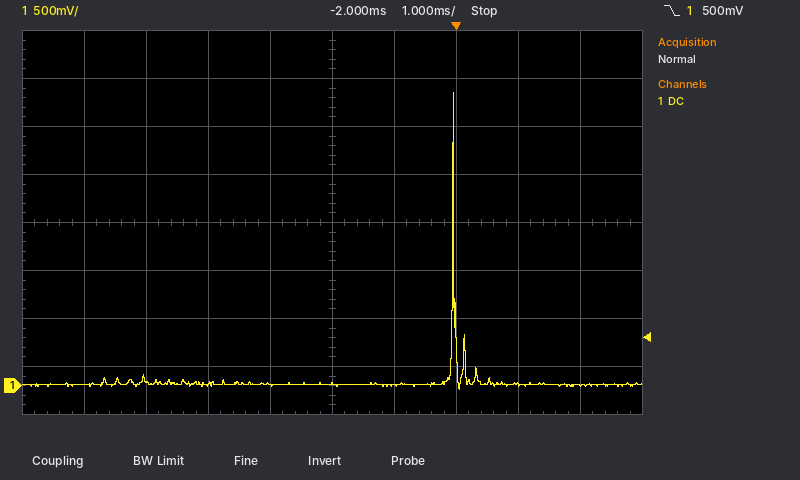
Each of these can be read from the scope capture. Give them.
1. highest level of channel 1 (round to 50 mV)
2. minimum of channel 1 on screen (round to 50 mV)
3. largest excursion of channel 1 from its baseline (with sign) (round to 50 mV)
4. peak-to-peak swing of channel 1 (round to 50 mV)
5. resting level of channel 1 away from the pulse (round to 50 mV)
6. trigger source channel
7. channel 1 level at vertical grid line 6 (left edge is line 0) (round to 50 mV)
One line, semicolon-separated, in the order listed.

3.05 V; -50 mV; +3.05 V; 3.10 V; 0 mV; channel 1; 0 mV
